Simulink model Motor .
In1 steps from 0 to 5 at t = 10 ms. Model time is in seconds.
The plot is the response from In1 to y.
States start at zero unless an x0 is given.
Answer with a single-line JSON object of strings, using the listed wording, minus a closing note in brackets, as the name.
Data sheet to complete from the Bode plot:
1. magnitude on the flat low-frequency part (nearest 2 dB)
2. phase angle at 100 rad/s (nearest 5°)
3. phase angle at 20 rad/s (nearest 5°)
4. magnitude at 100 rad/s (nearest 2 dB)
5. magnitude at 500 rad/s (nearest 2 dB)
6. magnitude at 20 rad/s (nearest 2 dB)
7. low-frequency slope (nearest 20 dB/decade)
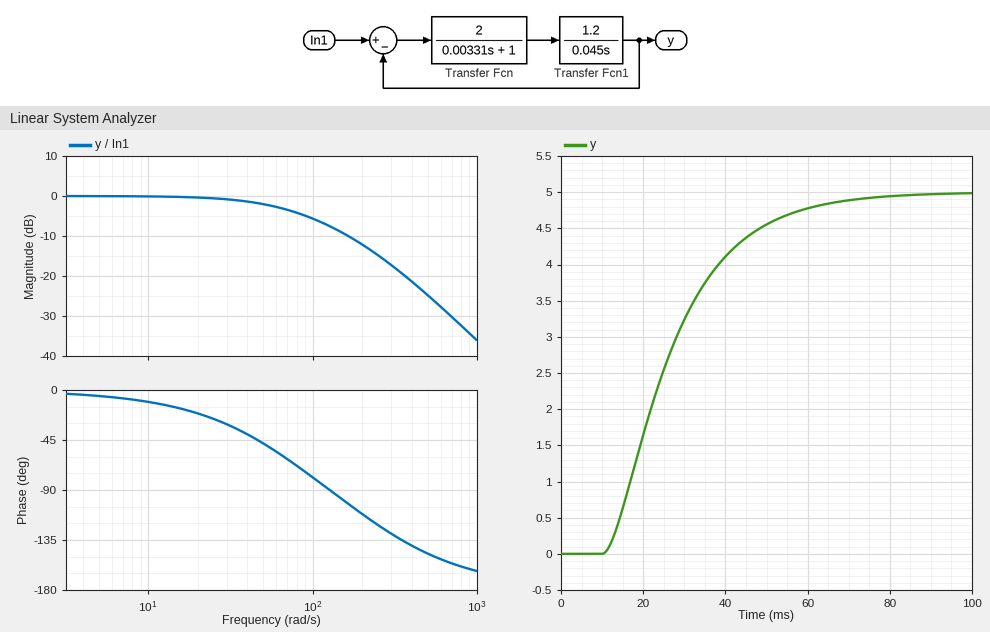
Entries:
{"magnitude on the flat low-frequency part": "0 dB", "phase angle at 100 rad/s": "-80°", "phase angle at 20 rad/s": "-20°", "magnitude at 100 rad/s": "-6 dB", "magnitude at 500 rad/s": "-24 dB", "magnitude at 20 rad/s": "0 dB", "low-frequency slope": "0 dB/decade"}
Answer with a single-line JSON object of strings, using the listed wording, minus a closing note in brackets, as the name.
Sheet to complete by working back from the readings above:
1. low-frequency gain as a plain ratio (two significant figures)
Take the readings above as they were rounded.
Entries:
{"low-frequency gain as a plain ratio": "1.0"}
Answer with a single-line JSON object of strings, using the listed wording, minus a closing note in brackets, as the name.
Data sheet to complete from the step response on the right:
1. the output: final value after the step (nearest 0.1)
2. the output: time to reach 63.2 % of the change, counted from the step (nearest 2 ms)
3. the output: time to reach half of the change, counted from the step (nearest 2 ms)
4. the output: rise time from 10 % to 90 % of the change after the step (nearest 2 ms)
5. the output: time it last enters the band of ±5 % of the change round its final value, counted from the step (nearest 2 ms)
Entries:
{"the output: final value after the step": "5.0", "the output: time to reach 63.2 % of the change, counted from the step": "20 ms", "the output: time to reach half of the change, counted from the step": "14 ms", "the output: rise time from 10 % to 90 % of the change after the step": "34 ms", "the output: time it last enters the band of ±5 % of the change round its final value, counted from the step": "48 ms"}
